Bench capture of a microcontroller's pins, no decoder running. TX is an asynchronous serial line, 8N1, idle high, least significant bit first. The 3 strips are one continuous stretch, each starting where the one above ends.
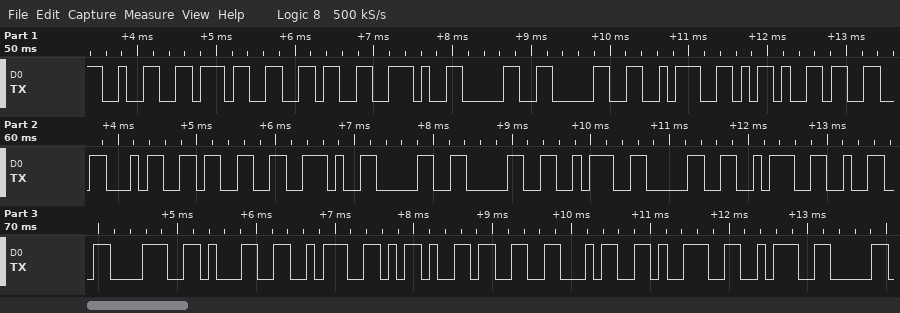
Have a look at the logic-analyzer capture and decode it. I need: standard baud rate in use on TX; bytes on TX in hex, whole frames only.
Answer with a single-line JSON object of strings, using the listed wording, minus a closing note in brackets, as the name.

{"standard baud rate in use on TX": "9600 baud", "bytes on TX in hex, whole frames only": "32 37 36 2E 30 30 3A 2D 33 34 33 2E 30 30 3A 30 3A 32 38 31 3A 2D 33 34 39 3A"}
